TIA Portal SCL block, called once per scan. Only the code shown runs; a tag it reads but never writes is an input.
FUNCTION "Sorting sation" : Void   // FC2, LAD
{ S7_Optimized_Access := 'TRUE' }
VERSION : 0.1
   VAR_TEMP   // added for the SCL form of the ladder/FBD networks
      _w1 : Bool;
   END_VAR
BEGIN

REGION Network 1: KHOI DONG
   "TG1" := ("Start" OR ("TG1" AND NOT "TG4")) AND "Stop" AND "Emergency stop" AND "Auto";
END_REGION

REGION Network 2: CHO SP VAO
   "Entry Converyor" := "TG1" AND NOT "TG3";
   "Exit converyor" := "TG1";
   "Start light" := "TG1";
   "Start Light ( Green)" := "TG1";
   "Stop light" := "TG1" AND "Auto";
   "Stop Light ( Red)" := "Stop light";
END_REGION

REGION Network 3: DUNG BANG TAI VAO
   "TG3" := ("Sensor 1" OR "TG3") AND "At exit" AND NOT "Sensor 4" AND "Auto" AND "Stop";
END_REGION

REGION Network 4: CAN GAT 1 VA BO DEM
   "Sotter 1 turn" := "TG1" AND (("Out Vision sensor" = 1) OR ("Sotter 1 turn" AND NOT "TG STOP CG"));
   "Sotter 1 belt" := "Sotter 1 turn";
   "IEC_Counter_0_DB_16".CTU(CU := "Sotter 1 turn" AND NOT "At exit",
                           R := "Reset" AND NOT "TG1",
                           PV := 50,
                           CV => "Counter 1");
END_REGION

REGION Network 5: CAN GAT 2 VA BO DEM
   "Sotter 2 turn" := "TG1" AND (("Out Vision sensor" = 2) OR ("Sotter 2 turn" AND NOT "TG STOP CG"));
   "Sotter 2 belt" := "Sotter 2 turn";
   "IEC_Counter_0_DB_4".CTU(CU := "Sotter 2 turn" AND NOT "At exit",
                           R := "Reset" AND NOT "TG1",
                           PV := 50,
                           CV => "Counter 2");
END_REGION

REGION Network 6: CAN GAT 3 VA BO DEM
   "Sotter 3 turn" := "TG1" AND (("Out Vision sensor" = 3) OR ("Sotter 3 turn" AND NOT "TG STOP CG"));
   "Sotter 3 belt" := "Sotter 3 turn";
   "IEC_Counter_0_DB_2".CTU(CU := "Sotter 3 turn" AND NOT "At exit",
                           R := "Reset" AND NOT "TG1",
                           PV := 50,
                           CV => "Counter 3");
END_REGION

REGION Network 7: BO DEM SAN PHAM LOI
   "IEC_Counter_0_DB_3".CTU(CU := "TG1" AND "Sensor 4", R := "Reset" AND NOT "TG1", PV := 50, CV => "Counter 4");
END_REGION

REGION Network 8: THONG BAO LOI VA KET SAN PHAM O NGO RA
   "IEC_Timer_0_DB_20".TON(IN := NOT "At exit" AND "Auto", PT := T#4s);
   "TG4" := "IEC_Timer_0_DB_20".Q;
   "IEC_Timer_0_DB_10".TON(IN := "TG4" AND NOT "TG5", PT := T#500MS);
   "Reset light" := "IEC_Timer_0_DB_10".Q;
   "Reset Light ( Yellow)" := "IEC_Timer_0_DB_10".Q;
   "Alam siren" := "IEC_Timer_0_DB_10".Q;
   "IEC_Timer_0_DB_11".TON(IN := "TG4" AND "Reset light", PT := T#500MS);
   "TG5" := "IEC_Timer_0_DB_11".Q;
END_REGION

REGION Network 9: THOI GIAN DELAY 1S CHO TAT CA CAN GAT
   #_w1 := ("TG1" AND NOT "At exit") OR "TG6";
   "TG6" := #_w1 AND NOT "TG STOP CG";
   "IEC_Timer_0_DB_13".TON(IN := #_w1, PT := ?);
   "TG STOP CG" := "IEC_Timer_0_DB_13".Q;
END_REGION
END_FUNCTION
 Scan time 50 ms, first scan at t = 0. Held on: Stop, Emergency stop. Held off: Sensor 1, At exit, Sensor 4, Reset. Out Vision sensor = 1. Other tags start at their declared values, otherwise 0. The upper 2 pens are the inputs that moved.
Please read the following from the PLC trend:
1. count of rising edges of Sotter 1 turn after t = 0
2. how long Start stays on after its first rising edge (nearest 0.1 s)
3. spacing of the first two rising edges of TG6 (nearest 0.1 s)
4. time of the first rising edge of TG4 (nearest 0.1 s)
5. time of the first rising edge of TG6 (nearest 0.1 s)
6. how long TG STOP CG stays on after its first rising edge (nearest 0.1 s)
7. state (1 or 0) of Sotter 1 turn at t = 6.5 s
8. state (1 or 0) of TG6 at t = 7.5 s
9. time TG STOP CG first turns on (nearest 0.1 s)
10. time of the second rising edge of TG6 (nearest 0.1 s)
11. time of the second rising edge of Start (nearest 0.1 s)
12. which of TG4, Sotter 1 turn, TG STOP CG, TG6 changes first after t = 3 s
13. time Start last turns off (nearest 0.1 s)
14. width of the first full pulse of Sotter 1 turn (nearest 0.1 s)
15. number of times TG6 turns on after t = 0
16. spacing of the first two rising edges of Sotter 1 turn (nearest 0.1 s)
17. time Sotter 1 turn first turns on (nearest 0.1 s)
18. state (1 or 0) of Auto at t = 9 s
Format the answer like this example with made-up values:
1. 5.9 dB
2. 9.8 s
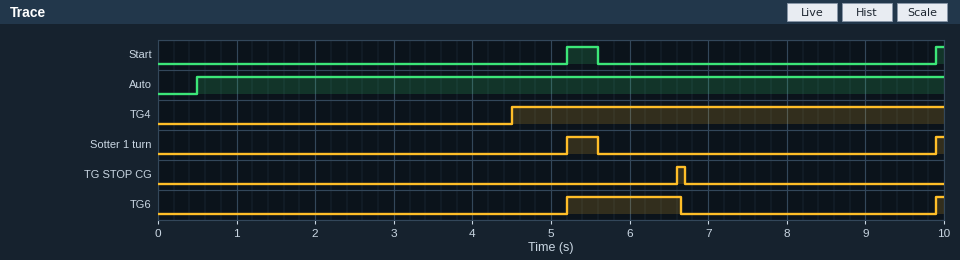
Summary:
1. 2
2. 0.4 s
3. 4.7 s
4. 4.5 s
5. 5.2 s
6. 0.1 s
7. 0
8. 0
9. 6.6 s
10. 9.9 s
11. 9.9 s
12. TG4
13. 5.6 s
14. 0.4 s
15. 2
16. 4.7 s
17. 5.2 s
18. 1
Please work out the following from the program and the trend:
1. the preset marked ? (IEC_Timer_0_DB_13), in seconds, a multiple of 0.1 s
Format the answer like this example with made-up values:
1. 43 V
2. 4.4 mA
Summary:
1. 1.4 s
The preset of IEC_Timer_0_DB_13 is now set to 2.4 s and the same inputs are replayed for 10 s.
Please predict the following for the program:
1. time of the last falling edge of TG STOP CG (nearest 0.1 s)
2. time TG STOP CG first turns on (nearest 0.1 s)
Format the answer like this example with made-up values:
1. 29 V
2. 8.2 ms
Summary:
1. 7.7 s
2. 7.6 s
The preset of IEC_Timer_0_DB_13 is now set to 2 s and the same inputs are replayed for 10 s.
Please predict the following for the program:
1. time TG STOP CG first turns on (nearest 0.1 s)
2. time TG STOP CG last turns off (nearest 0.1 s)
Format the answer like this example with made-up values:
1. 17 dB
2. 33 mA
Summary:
1. 7.2 s
2. 7.3 s
